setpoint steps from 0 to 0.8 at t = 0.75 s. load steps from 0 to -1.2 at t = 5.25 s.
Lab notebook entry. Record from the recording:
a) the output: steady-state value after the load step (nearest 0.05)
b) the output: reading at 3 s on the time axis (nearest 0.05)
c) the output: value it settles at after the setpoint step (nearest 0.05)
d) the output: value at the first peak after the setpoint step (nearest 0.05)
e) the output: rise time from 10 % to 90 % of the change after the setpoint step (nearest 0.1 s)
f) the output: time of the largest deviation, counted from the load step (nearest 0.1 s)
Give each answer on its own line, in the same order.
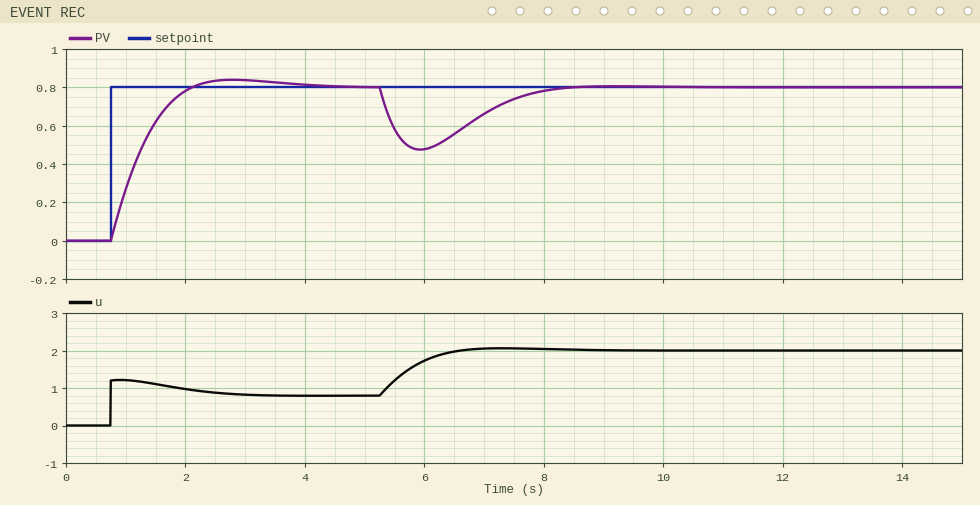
0.80
0.85
0.80
0.85
0.9 s
0.7 s
